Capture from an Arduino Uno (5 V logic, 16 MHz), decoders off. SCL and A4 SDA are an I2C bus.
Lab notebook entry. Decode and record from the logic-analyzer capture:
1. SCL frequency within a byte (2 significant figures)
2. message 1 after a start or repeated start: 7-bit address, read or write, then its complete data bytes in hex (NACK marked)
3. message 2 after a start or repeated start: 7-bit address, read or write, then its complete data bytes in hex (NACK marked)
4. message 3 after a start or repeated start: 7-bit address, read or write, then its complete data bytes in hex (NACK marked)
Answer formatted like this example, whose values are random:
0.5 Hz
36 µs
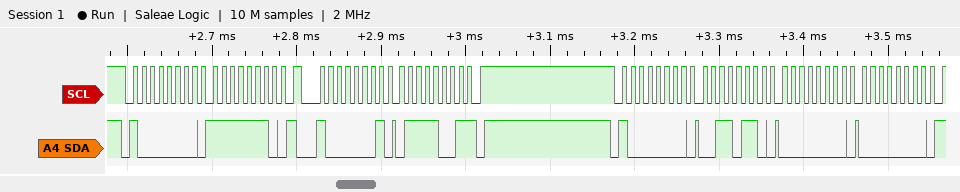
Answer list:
100 kHz
0x40 write: FE
0x40 read: 79 NACK
0x40 write: 36 00 00
